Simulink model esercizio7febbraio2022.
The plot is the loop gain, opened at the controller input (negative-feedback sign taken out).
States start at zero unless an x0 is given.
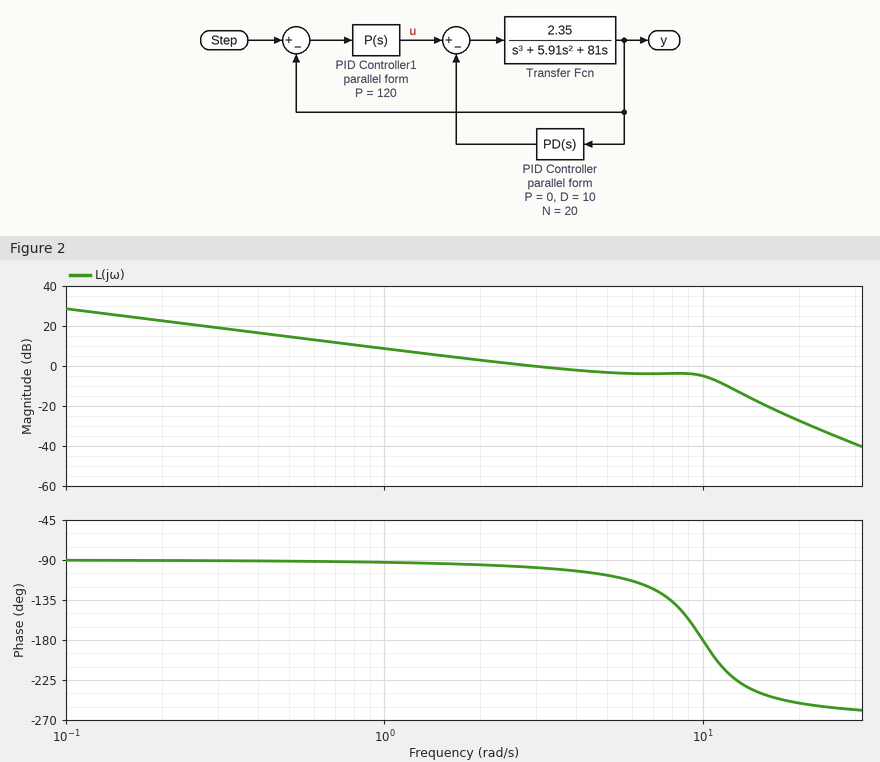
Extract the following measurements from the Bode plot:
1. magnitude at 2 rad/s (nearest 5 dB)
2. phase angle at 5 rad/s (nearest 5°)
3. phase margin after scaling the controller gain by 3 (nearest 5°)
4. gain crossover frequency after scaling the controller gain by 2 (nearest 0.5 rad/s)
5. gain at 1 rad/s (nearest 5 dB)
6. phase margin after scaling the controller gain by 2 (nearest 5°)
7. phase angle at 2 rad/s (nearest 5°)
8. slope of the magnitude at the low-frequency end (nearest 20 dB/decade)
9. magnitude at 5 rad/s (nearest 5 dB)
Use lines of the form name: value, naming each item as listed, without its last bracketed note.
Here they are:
magnitude at 2 rad/s: 5 dB
phase angle at 5 rad/s: -105°
phase margin after scaling the controller gain by 3: -35°
gain crossover frequency after scaling the controller gain by 2: 10.5 rad/s
gain at 1 rad/s: 10 dB
phase margin after scaling the controller gain by 2: -10°
phase angle at 2 rad/s: -95°
slope of the magnitude at the low-frequency end: -20 dB/decade
magnitude at 5 rad/s: -5 dB
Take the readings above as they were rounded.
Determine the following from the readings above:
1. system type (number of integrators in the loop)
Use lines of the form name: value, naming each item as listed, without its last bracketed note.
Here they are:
system type: 1
